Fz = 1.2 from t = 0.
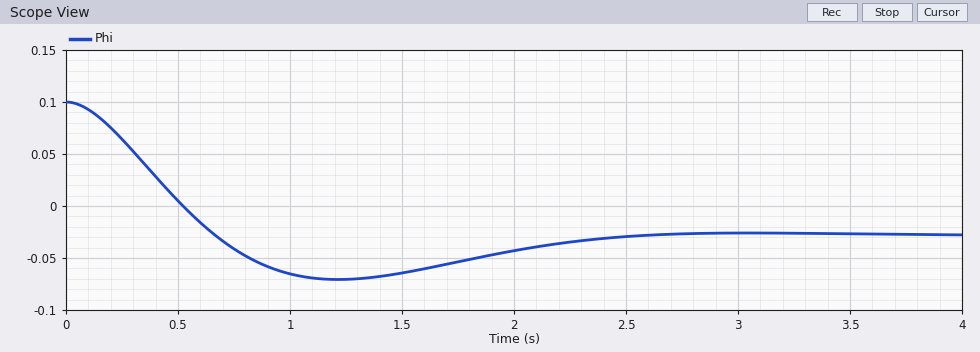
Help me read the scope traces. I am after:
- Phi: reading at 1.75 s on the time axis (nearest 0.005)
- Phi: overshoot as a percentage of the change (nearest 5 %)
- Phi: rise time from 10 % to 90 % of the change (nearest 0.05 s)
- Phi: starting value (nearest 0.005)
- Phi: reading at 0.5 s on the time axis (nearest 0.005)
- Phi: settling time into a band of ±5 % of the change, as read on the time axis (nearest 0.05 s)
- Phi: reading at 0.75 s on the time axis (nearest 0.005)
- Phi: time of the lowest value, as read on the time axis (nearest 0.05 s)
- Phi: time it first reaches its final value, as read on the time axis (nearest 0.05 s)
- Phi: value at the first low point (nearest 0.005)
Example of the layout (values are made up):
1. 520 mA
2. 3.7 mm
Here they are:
1. -0.055
2. 35 %
3. 0.45 s
4. 0.100
5. 0.005
6. 2.30 s
7. -0.040
8. 1.20 s
9. 0.65 s
10. -0.070
